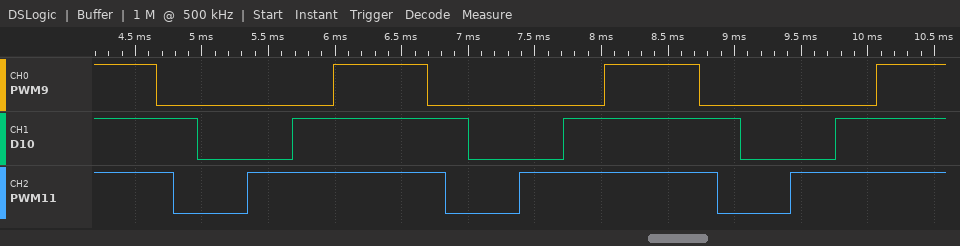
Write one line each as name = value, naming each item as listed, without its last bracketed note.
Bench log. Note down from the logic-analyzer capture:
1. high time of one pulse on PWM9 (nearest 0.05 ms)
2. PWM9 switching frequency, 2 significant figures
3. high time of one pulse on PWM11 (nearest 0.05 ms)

high time of one pulse on PWM9 = 0.70 ms
PWM9 switching frequency, 2 significant figures = 490 Hz
high time of one pulse on PWM11 = 1.50 ms
